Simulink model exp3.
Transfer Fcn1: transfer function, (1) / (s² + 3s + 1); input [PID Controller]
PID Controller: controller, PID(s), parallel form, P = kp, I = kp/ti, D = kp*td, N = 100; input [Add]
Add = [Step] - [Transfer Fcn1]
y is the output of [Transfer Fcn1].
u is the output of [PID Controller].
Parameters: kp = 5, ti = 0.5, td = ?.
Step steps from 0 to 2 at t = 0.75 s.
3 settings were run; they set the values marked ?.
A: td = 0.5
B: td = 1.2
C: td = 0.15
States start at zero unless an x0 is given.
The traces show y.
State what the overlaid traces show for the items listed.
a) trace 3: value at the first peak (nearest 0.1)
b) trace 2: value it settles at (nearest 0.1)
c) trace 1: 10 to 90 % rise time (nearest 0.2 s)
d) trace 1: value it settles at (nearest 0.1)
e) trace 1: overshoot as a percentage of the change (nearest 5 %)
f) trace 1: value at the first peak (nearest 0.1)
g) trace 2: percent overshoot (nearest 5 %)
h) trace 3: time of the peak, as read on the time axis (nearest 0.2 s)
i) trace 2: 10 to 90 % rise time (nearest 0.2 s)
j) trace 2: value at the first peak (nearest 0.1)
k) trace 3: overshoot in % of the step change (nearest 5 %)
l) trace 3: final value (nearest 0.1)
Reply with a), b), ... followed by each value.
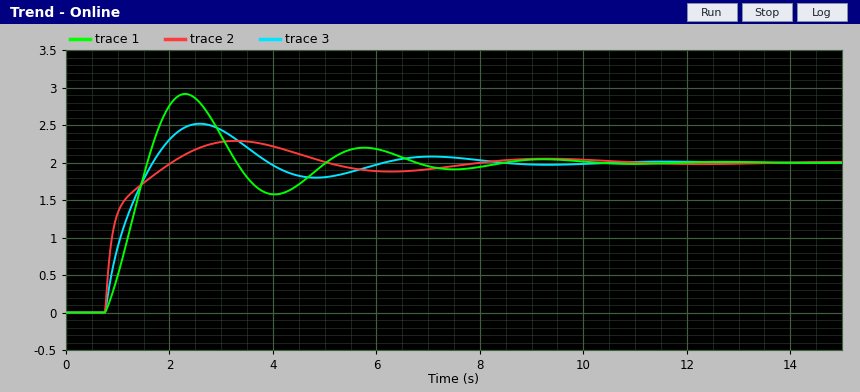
a) 2.5
b) 2.0
c) 0.6 s
d) 2.0
e) 45 %
f) 2.9
g) 15 %
h) 2.6 s
i) 0.8 s
j) 2.3
k) 25 %
l) 2.0
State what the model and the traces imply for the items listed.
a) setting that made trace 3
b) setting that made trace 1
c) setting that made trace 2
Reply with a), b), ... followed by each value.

a) A
b) C
c) B
